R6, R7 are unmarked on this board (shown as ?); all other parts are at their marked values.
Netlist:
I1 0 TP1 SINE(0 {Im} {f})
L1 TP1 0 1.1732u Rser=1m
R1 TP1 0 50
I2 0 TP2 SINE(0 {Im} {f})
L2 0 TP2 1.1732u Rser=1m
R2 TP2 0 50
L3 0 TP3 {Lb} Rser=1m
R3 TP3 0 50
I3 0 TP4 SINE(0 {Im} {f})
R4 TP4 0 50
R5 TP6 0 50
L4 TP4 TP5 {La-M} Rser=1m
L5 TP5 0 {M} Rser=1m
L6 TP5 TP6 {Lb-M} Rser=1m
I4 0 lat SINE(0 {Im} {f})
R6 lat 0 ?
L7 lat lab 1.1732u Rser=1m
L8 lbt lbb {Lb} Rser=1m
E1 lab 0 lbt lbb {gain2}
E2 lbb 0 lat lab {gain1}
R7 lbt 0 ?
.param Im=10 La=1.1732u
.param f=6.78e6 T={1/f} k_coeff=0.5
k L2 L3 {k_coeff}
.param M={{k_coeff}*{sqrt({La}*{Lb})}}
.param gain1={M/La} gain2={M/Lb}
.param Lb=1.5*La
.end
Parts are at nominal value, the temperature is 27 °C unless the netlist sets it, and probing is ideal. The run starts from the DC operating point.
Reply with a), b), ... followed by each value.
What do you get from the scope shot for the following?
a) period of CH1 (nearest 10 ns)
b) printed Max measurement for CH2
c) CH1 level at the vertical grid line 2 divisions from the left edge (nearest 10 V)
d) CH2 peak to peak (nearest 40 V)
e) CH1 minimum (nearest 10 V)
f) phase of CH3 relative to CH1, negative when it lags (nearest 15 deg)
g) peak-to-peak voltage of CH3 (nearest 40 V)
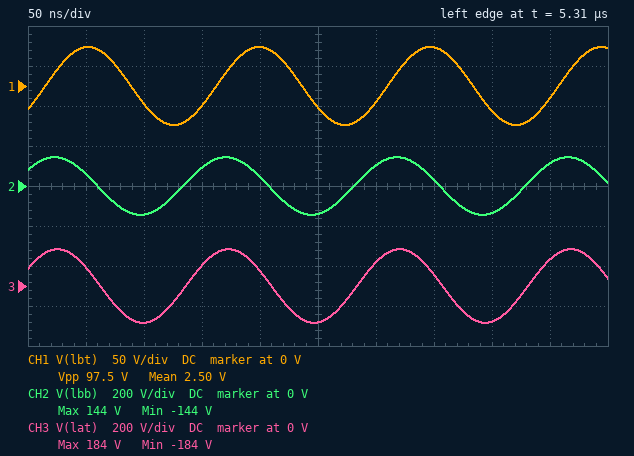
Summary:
a) 150 ns
b) 144 V
c) -20 V
d) 280 V
e) -50 V
f) 60 deg
g) 360 V
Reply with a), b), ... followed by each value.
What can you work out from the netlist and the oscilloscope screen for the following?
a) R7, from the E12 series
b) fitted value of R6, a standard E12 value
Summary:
a) 27 Ω
b) 22 Ω
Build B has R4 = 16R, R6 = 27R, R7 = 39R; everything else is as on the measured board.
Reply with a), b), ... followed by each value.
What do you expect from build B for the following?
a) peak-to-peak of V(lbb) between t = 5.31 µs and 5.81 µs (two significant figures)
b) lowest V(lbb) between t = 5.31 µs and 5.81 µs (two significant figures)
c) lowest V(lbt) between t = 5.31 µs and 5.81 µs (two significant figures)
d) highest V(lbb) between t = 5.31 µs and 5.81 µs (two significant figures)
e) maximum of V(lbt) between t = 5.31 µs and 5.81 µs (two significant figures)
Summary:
a) 320 V
b) -160 V
c) -74 V
d) 160 V
e) 74 V
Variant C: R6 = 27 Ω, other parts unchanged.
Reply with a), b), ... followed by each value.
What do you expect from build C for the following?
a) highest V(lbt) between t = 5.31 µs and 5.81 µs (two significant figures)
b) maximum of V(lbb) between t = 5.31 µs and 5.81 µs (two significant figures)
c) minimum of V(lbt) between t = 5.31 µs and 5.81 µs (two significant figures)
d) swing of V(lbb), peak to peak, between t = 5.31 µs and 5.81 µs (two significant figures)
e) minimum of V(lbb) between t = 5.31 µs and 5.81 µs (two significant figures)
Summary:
a) 56 V
b) 170 V
c) -56 V
d) 330 V
e) -170 V
